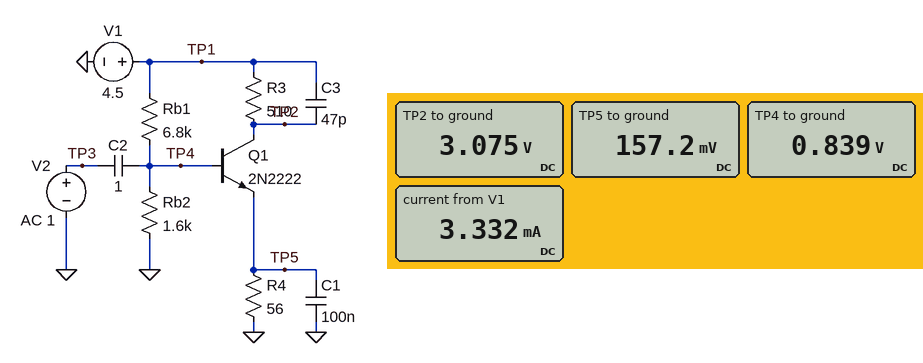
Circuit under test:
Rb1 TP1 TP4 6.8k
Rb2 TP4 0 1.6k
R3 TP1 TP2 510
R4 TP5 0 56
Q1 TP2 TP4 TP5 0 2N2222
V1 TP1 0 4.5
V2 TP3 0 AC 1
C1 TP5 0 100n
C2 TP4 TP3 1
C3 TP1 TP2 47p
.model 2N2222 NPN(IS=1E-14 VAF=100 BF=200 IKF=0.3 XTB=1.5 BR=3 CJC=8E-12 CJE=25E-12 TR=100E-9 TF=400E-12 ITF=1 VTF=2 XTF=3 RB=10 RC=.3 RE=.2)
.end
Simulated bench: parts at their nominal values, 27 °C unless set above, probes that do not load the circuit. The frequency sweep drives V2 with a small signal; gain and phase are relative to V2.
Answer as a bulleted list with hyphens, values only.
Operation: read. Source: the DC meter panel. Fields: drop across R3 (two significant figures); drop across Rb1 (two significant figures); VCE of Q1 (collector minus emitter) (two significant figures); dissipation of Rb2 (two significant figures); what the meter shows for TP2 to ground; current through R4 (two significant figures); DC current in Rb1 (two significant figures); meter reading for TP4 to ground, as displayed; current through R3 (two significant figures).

- 1.4 V
- 3.7 V
- 2.9 V
- 440 µW
- 3.075 V
- 2.8 mA
- 540 µA
- 0.839 V
- 2.8 mA
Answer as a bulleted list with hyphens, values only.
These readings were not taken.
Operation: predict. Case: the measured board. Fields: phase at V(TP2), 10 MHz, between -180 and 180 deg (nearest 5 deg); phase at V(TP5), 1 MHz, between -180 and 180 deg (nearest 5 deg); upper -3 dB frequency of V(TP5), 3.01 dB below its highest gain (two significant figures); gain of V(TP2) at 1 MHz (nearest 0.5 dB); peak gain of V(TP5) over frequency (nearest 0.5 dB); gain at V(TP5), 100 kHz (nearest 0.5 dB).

- 115 deg
- -80 deg
- 190 kHz
- 34.0 dB
- -1.5 dB
- -2.5 dB
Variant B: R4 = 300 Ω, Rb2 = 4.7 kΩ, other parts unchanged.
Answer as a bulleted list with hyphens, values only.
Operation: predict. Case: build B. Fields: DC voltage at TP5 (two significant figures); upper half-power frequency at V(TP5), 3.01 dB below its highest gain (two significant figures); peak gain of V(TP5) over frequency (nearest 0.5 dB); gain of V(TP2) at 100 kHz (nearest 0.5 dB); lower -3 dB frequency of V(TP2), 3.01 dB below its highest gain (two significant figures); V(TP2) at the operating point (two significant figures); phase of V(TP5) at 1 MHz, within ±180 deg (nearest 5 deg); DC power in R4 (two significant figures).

- 1.1 V
- 220 kHz
- 0 dB
- 29.0 dB
- 200 kHz
- 2.6 V
- -80 deg
- 4.0 mW
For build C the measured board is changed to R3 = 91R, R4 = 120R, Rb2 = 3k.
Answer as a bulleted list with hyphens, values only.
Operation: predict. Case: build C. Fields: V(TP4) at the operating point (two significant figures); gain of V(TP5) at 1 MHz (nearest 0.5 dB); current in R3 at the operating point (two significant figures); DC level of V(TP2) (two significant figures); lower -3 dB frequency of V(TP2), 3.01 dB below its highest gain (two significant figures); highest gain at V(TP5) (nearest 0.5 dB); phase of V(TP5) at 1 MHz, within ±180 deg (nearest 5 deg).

- 1.3 V
- -11.0 dB
- 5.2 mA
- 4.0 V
- 310 kHz
- -0.5 dB
- -75 deg
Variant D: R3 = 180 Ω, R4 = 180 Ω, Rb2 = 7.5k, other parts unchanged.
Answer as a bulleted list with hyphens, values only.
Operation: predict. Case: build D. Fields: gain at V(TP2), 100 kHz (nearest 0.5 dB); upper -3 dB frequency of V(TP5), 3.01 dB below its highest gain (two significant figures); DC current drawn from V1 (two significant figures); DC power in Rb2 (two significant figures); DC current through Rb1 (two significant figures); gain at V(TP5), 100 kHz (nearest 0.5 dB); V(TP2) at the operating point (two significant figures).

- 20.5 dB
- 470 kHz
- 8.6 mA
- 650 µW
- 340 µA
- -0.5 dB
- 3.0 V
